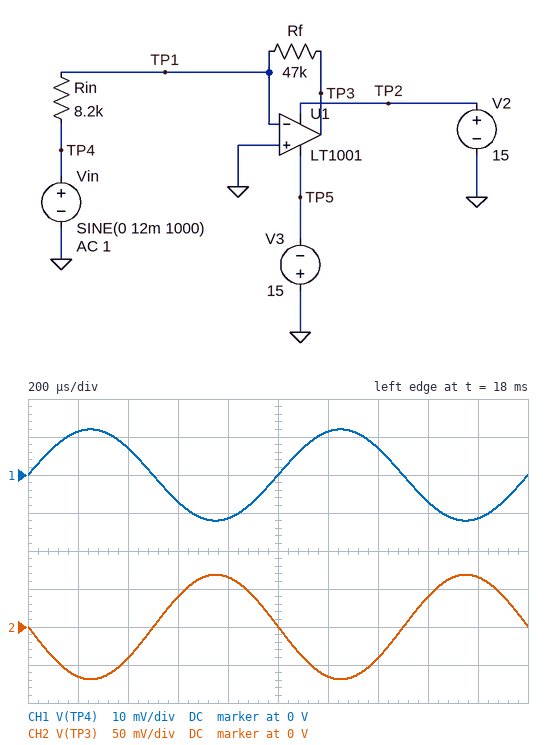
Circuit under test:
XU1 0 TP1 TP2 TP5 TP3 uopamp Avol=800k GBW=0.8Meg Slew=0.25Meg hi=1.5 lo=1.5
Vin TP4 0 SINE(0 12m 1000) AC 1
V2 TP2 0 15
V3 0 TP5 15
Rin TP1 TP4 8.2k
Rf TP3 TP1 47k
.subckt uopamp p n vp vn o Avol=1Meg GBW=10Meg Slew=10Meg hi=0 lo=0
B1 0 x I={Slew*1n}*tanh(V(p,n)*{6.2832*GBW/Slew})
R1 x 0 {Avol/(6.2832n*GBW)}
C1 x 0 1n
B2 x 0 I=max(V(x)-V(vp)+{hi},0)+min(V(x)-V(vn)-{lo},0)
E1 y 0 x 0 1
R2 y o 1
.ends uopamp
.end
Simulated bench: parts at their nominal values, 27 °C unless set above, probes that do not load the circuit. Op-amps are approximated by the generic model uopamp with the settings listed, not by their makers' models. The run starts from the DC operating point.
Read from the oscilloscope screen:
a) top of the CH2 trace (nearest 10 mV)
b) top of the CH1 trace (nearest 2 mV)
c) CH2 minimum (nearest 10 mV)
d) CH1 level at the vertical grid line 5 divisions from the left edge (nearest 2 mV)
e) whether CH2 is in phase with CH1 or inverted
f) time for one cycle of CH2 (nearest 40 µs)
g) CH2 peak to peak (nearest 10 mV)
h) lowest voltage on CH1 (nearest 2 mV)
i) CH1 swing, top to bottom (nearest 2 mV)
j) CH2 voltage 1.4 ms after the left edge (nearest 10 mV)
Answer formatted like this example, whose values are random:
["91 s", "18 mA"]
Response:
["70 mV", "12 mV", "-70 mV", "0 V", "inverted", "1.00 ms", "140 mV", "-12 mV", "24 mV", "-40 mV"]
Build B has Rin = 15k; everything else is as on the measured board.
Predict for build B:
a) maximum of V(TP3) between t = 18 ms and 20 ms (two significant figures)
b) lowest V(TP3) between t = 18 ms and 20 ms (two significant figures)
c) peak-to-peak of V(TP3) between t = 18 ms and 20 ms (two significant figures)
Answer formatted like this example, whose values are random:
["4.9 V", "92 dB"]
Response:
["38 mV", "-38 mV", "75 mV"]
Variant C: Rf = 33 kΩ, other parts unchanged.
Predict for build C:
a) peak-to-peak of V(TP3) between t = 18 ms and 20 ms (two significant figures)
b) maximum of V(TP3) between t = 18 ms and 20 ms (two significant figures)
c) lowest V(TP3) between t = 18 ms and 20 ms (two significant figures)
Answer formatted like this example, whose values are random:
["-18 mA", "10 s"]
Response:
["97 mV", "48 mV", "-48 mV"]
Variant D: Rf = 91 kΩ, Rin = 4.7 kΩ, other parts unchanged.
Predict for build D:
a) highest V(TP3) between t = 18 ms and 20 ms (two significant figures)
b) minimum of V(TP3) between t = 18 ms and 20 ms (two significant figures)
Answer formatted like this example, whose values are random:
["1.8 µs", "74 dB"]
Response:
["230 mV", "-230 mV"]
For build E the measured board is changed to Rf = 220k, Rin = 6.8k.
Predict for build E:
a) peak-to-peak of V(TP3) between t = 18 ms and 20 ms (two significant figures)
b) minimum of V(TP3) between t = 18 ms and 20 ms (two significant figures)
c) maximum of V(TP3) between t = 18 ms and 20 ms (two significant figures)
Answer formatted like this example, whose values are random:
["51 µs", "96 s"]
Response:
["780 mV", "-390 mV", "390 mV"]
